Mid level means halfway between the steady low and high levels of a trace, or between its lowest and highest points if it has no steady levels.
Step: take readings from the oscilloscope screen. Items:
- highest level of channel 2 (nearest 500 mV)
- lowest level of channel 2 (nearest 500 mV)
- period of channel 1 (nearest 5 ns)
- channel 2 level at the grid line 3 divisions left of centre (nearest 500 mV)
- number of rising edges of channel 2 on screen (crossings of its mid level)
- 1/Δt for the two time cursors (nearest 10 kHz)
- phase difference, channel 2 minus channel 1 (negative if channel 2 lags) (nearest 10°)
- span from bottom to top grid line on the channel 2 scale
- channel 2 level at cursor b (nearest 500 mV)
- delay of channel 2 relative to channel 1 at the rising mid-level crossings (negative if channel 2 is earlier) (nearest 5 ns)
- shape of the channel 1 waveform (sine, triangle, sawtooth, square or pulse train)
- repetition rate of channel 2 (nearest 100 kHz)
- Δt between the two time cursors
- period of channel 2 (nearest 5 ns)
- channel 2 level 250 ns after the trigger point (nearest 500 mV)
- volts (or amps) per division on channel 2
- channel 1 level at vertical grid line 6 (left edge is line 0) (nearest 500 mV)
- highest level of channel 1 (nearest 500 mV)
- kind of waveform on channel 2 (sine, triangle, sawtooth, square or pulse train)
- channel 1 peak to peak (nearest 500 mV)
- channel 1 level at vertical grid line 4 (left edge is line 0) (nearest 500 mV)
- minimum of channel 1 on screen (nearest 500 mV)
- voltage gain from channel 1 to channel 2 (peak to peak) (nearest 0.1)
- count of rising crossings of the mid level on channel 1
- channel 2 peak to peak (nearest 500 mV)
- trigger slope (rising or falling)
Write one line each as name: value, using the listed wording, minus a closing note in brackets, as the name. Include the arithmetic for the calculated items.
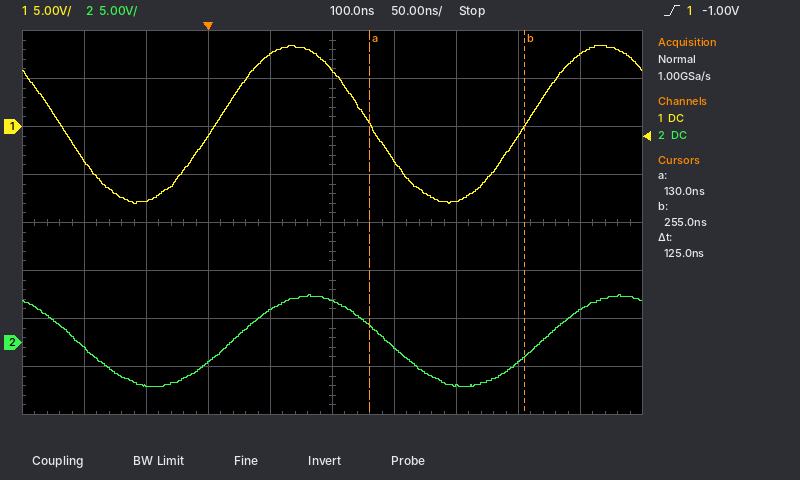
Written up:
highest level of channel 2: 5.0 V
lowest level of channel 2: -4.5 V
period of channel 1: 250 ns
channel 2 level at the grid line 3 divisions left of centre: -4.5 V
number of rising edges of channel 2 on screen: 2
1/Δt for the two time cursors: 1 / 125 ns ≈ 8.00 MHz
phase difference, channel 2 minus channel 1 (negative if channel 2 lags): −360° × (+15 ns) / 250 ns ≈ -21.6°, so -20° to the nearest 10°
span from bottom to top grid line on the channel 2 scale: 40 V
channel 2 level at cursor b: -1.5 V
delay of channel 2 relative to channel 1 at the rising mid-level crossings (negative if channel 2 is earlier): +15 ns
shape of the channel 1 waveform: sine
repetition rate of channel 2: 1 / 250 ns ≈ 4.0 MHz
Δt between the two time cursors: 125 ns
period of channel 2: 250 ns
channel 2 level 250 ns after the trigger point: -2.0 V
volts (or amps) per division on channel 2: 5 V
channel 1 level at vertical grid line 6 (left edge is line 0): -3.5 V
highest level of channel 1: 8.5 V
kind of waveform on channel 2: sine
channel 1 peak to peak: 8.5 V − (-8.0 V) = 16.5 V
channel 1 level at vertical grid line 4 (left edge is line 0): 7.5 V
minimum of channel 1 on screen: -8.0 V
voltage gain from channel 1 to channel 2 (peak to peak): 9.5 V / 16.5 V ≈ 0.6
count of rising crossings of the mid level on channel 1: 2
channel 2 peak to peak: 5.0 V − (-4.5 V) = 9.5 V
trigger slope: rising
